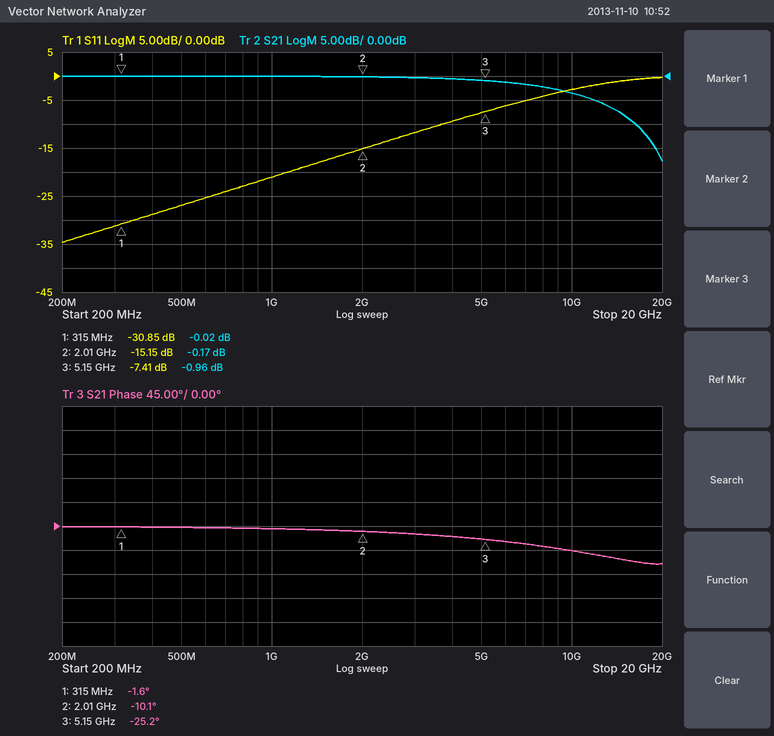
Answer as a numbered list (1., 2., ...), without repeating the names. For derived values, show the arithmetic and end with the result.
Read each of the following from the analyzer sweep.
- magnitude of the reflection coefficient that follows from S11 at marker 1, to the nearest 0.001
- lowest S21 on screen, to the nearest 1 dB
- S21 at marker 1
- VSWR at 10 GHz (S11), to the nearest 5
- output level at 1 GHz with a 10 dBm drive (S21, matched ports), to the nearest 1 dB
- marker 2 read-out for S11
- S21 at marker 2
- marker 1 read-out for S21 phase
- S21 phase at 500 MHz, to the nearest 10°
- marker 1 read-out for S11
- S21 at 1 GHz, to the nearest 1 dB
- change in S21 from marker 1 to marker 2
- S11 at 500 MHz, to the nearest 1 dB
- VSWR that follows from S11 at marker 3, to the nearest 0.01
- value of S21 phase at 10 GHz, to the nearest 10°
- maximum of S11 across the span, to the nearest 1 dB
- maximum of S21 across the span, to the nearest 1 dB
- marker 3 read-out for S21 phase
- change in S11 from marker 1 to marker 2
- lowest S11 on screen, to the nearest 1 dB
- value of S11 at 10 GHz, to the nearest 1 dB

1. 10^(-30.85/20) ≈ 0.029
2. -18 dB
3. -0.02 dB
4. |Γ| = 10^(-3/20) = 0.7079; VSWR = (1 + 0.7079)/(1 − 0.7079) ≈ 5.85, so 5 to the nearest 5
5. 10 dBm + (0 dB) = 10 dBm
6. -15.15 dB
7. -0.17 dB
8. -1.6°
9. 0°
10. -30.85 dB
11. 0 dB
12. -0.17 − (-0.02) = -0.15 dB
13. -27 dB
14. (1 + 0.4261)/(1 − 0.4261) ≈ 2.48
15. -50°
16. 0 dB
17. 0 dB
18. -25.2°
19. -15.15 − (-30.85) = 15.70 dB
20. -35 dB
21. -3 dB
